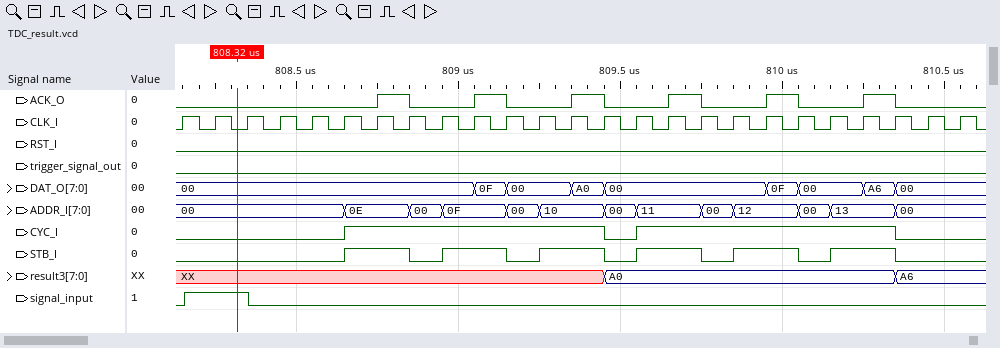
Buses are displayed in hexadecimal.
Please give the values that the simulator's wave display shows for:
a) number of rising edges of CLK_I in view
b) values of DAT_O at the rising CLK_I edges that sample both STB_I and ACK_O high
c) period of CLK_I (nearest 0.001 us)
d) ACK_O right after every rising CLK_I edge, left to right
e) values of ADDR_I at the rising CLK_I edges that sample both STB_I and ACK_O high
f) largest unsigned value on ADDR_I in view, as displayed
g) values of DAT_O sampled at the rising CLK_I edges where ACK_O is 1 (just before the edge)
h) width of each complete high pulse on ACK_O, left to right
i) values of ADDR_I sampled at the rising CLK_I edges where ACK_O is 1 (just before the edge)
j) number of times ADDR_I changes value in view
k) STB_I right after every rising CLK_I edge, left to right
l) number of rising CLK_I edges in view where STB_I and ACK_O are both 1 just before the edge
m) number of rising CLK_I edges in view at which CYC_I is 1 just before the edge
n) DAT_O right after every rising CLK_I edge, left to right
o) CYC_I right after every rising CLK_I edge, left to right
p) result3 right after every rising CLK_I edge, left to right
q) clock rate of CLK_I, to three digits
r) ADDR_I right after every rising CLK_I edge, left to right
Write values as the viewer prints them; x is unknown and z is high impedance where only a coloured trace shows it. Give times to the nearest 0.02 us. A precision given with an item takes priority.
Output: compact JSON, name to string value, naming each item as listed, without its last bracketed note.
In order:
{"number of rising edges of CLK_I in view": "25", "values of DAT_O at the rising CLK_I edges that sample both STB_I and ACK_O high": "00, 0F, A0, 00, 0F, A6", "period of CLK_I": "0.1 us", "ACK_O right after every rising CLK_I edge, left to right": "0 0 0 0 0 0 1 0 0 1 0 0 1 0 0 1 0 0 1 0 0 1 0 0 0", "values of ADDR_I at the rising CLK_I edges that sample both STB_I and ACK_O high": "0E, 0F, 10, 11, 12, 13", "largest unsigned value on ADDR_I in view, as displayed": "13", "values of DAT_O sampled at the rising CLK_I edges where ACK_O is 1": "00, 0F, A0, 00, 0F, A6", "width of each complete high pulse on ACK_O, left to right": "0.1 us, 0.1 us, 0.1 us, 0.1 us, 0.1 us, 0.1 us", "values of ADDR_I sampled at the rising CLK_I edges where ACK_O is 1": "0E, 0F, 10, 11, 12, 13", "number of times ADDR_I changes value in view": "12", "STB_I right after every rising CLK_I edge, left to right": "0 0 0 0 0 1 1 0 1 1 0 1 1 0 1 1 0 1 1 0 1 1 0 0 0", "number of rising CLK_I edges in view where STB_I and ACK_O are both 1 just before the edge": "6", "number of rising CLK_I edges in view at which CYC_I is 1 just before the edge": "16", "DAT_O right after every rising CLK_I edge, left to right": "00, 00, 00, 00, 00, 00, 00, 00, 00, 0F, 00, 00, A0, 00, 00, 00, 00, 00, 0F, 00, 00, A6, 00, 00, 00", "CYC_I right after every rising CLK_I edge, left to right": "0 0 0 0 0 1 1 1 1 1 1 1 1 0 1 1 1 1 1 1 1 1 0 0 0", "result3 right after every rising CLK_I edge, left to right": "XX, XX, XX, XX, XX, XX, XX, XX, XX, XX, XX, XX, XX, A0, A0, A0, A0, A0, A0, A0, A0, A0, A6, A6, A6", "clock rate of CLK_I, to three digits": "10.0 MHz", "ADDR_I right after every rising CLK_I edge, left to right": "00, 00, 00, 00, 00, 0E, 0E, 00, 0F, 0F, 00, 10, 10, 00, 11, 11, 00, 12, 12, 00, 13, 13, 00, 00, 00"}
